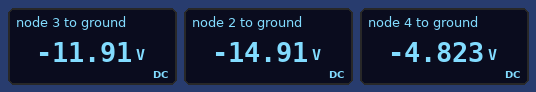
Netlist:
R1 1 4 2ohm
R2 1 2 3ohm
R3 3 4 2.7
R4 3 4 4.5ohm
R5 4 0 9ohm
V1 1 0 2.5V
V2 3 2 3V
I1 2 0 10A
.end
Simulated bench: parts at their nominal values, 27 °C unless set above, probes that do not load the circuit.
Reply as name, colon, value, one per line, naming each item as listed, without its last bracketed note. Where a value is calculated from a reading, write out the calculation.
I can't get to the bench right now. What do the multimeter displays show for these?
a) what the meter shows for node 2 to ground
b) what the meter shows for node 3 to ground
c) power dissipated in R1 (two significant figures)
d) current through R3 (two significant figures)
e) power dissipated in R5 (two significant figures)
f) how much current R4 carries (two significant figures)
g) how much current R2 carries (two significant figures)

what the meter shows for node 2 to ground: -14.91 V
what the meter shows for node 3 to ground: -11.91 V
power dissipated in R1: (2.5 V - (-4.823 V))^2 / 2 Ω = 27 W
current through R3: (-4.823 V - (-11.91 V)) / 2.7 Ω = 2.6 A
power dissipated in R5: (0 V - (-4.823 V))^2 / 9 Ω = 2.6 W
how much current R4 carries: (-4.823 V - (-11.91 V)) / 4.5 Ω = 1.6 A
how much current R2 carries: (2.5 V - (-14.91 V)) / 3 Ω = 5.8 A
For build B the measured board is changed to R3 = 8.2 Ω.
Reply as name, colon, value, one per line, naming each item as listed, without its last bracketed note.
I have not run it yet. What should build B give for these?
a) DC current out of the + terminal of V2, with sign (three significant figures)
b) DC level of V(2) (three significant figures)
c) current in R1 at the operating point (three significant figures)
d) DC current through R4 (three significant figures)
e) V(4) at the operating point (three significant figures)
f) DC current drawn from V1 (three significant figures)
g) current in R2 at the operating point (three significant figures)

DC current out of the + terminal of V2, with sign: -3.52 A
DC level of V(2): -16.9 V
current in R1 at the operating point: 3.11 A
DC current through R4: 2.27 A
V(4) at the operating point: -3.71 V
DC current drawn from V1: 9.59 A
current in R2 at the operating point: 6.48 A
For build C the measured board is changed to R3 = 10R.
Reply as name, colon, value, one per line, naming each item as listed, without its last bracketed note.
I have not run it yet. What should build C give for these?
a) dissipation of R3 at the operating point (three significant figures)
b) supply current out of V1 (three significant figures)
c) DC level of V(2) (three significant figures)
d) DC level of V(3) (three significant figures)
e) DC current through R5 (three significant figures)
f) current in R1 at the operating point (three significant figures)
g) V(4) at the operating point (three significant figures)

dissipation of R3 at the operating point: 11.3 W
supply current out of V1: 9.60 A
DC level of V(2): -17.2 V
DC level of V(3): -14.2 V
DC current through R5: 396 mA
current in R1 at the operating point: 3.03 A
V(4) at the operating point: -3.57 V
